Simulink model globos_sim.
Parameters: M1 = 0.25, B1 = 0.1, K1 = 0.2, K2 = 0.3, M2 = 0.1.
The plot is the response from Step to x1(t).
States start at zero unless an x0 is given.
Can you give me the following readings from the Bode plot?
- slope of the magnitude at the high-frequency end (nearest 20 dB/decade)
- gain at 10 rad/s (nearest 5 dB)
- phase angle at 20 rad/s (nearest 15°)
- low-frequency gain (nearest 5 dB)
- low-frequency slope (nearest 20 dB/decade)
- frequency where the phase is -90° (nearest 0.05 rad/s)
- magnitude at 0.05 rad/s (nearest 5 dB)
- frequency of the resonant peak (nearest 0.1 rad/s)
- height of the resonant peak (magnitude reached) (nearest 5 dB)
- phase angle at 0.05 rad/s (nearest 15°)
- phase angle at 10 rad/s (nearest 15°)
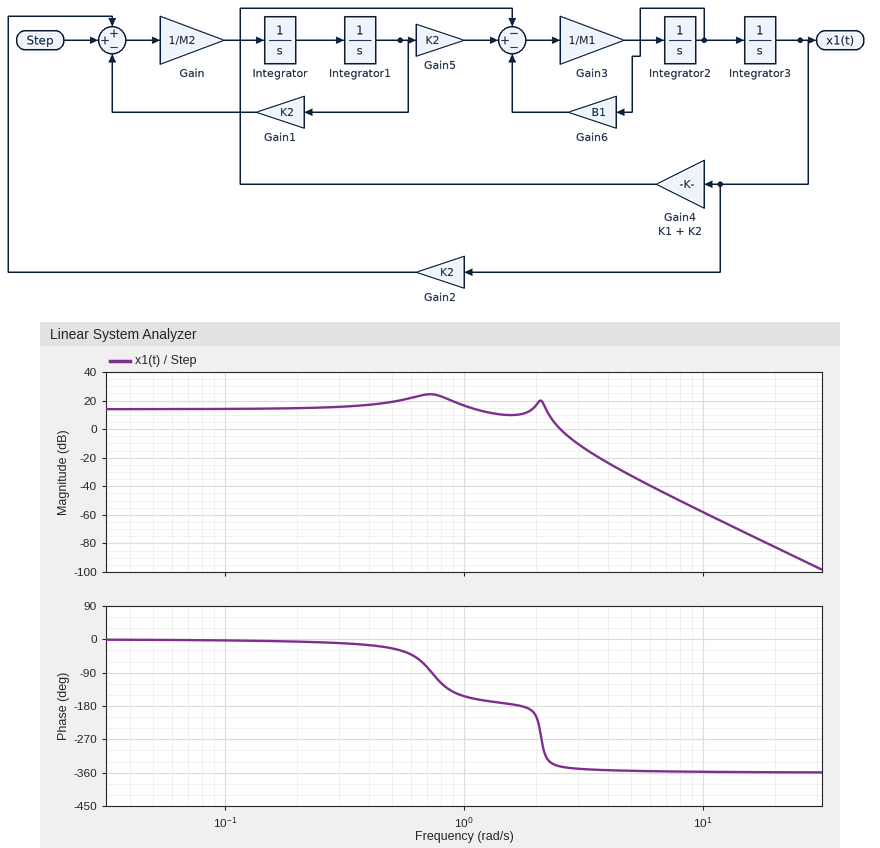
-80 dB/decade
-60 dB
-360°
15 dB
0 dB/decade
0.75 rad/s
15 dB
0.7 rad/s
25 dB
0°
-360°
